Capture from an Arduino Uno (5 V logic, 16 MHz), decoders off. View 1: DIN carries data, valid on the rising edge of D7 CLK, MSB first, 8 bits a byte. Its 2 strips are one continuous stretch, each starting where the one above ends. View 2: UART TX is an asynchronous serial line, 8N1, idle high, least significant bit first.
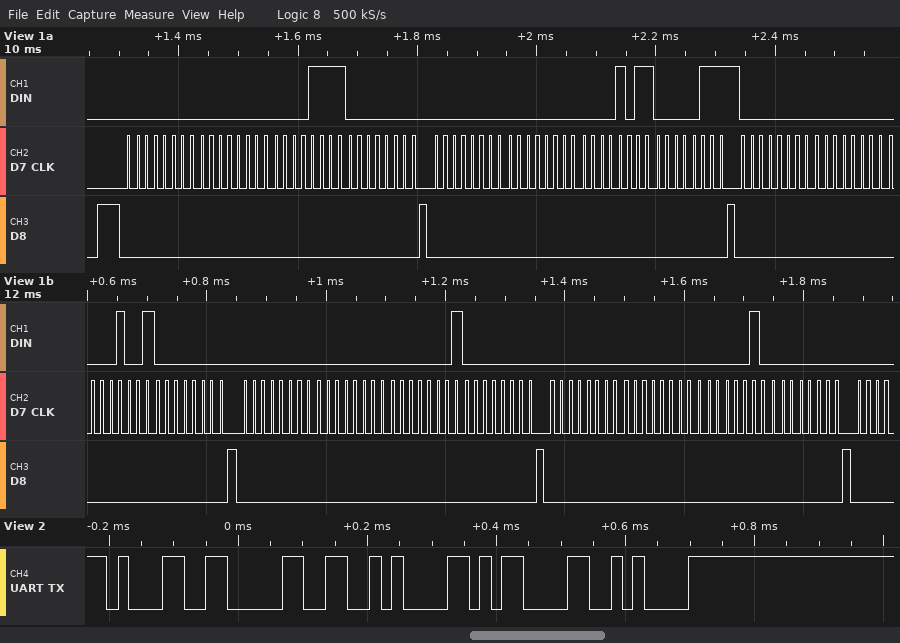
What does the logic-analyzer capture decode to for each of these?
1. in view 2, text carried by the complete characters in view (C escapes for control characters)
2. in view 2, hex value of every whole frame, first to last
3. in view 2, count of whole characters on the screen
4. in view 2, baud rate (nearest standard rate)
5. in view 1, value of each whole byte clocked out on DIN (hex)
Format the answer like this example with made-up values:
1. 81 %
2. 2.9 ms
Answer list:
1. "10\n\r\n"
2. 0x31 0x30 0x0A 0x0D 0x0A
3. 5
4. 57600 baud
5. 00 00 0F 00 00 00 0B 07 00 00 09 00 00 00 01 00 00 00 02 00
